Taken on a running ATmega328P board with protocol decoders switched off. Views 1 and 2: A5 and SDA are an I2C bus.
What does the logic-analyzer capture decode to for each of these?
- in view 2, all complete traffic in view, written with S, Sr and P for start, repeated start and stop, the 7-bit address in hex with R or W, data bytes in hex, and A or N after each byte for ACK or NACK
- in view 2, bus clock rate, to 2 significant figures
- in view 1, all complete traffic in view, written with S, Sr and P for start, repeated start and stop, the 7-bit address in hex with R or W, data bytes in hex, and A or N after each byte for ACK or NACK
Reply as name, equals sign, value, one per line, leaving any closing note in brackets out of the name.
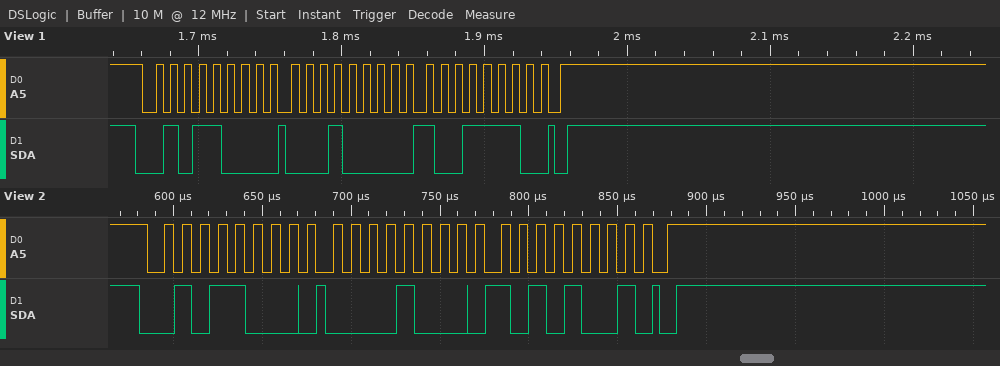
in view 2, all complete traffic in view, written with S, Sr and P for start, repeated start and stop, the 7-bit address in hex with R or W, data bytes in hex, and A or N after each byte for ACK or NACK = S 2CW A 08 A A9 A P
in view 2, bus clock rate, to 2 significant figures = 100 kHz
in view 1, all complete traffic in view, written with S, Sr and P for start, repeated start and stop, the 7-bit address in hex with R or W, data bytes in hex, and A or N after each byte for ACK or NACK = S 2CW A 10 A 9E A P
